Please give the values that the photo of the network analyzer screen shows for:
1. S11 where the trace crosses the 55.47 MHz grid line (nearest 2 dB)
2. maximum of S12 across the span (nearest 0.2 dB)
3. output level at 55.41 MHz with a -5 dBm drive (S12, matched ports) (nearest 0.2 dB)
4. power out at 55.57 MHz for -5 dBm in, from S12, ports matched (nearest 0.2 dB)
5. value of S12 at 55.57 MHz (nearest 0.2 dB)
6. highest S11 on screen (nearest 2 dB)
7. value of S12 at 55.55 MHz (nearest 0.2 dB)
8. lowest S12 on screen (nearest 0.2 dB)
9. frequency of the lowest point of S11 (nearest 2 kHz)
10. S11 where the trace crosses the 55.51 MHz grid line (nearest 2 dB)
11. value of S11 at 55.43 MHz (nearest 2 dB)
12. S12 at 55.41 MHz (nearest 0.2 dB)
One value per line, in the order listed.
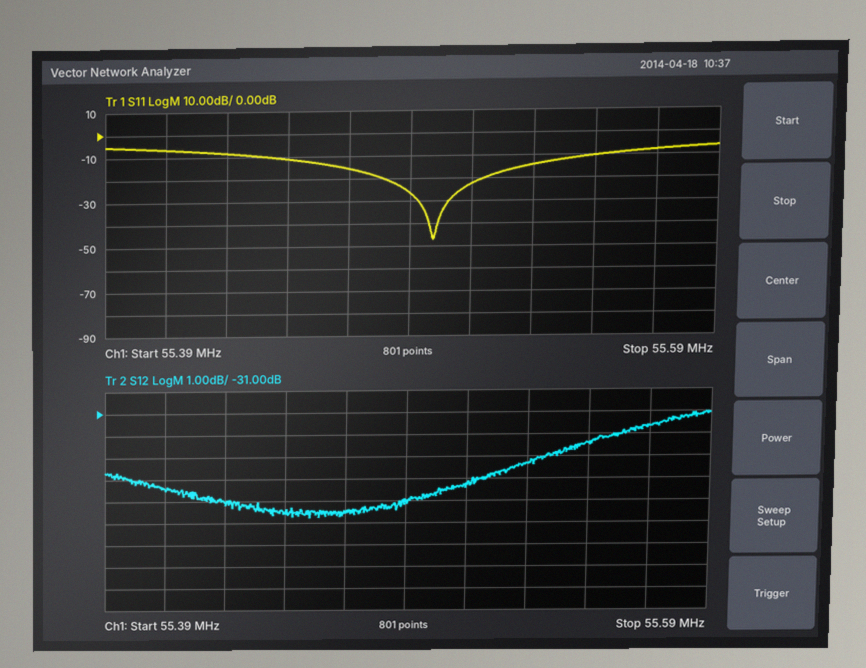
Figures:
-16 dB
-31.0 dB
-39.4 dBm
-36.6 dBm
-31.6 dB
-6 dB
-32.4 dB
-35.8 dB
55.498 MHz
-22 dB
-8 dB
-34.4 dB
